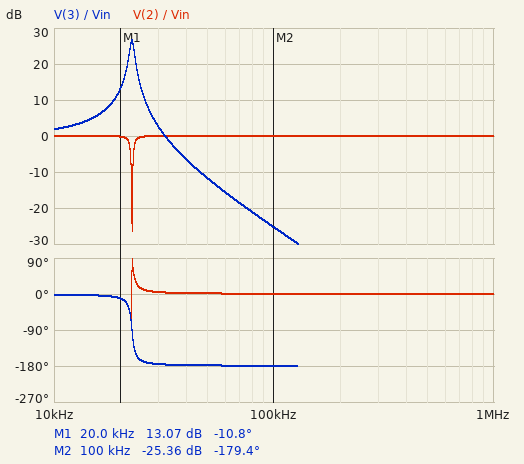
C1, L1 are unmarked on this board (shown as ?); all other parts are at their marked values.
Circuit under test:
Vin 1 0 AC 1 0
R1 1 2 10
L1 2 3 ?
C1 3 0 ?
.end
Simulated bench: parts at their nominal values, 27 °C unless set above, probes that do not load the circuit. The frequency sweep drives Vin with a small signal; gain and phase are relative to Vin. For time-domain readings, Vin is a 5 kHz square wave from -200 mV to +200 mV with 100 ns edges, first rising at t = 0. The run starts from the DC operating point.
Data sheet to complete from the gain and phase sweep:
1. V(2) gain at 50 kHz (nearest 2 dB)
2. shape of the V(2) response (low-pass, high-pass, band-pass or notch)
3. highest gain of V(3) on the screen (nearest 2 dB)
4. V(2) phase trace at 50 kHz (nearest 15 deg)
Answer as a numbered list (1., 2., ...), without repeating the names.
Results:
1. 0 dB
2. notch
3. 26 dB
4. 0 deg
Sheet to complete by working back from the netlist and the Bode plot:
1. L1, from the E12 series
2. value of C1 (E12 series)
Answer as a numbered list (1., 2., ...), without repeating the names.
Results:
1. 1.5 mH
2. 33 nF
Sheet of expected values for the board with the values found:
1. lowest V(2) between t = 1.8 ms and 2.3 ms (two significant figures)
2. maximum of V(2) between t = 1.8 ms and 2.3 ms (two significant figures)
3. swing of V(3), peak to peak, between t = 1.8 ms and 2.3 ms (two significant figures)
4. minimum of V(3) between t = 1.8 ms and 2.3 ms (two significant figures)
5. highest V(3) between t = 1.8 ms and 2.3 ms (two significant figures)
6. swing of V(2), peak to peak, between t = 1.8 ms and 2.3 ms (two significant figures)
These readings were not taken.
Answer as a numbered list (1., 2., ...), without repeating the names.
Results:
1. -210 mV
2. 210 mV
3. 1.0 V
4. -510 mV
5. 510 mV
6. 430 mV
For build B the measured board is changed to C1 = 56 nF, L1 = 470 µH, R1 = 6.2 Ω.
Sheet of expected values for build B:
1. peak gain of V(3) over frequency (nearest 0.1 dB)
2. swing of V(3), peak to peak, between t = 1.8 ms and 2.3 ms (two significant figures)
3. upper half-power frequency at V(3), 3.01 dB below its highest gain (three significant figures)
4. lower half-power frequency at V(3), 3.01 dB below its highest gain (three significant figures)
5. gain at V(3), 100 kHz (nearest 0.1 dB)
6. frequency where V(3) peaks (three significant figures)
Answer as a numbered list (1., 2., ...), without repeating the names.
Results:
1. 23.4 dB
2. 890 mV
3. 32.0 kHz
4. 29.9 kHz
5. -19.5 dB
6. 31.0 kHz
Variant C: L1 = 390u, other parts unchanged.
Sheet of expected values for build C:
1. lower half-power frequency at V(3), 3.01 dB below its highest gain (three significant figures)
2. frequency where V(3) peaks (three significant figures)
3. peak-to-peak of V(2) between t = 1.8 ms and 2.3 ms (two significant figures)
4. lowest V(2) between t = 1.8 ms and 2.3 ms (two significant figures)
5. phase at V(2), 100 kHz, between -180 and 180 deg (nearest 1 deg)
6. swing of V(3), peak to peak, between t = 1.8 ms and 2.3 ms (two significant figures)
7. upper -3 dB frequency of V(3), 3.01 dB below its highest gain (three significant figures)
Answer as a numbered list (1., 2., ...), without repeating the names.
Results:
1. 42.2 kHz
2. 44.3 kHz
3. 480 mV
4. -240 mV
5. 3 deg
6. 1.3 V
7. 46.3 kHz
